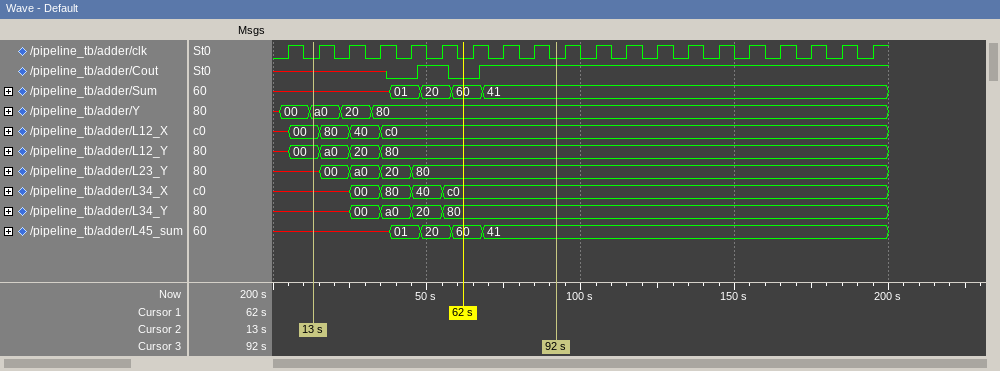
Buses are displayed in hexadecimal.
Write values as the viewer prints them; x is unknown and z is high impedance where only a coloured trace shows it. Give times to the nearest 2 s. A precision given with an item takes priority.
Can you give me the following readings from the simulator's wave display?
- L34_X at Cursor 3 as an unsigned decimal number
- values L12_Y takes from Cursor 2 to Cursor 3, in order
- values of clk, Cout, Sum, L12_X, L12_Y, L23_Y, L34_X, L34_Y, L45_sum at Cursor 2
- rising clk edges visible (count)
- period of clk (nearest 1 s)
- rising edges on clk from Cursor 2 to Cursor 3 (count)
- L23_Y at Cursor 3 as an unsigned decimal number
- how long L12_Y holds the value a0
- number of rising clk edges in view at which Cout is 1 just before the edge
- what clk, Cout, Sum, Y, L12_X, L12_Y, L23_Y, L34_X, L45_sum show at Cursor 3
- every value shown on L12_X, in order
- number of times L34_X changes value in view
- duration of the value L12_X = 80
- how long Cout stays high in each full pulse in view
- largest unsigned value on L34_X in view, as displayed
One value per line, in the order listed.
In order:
192
00, a0, 20, 80
clk=0, Cout=x, Sum=x, L12_X=00, L12_Y=00, L23_Y=x, L34_X=x, L34_Y=x, L45_sum=x
20
10 s
8
128
10 s
14
clk=0, Cout=1, Sum=41, Y=80, L12_X=c0, L12_Y=80, L23_Y=80, L34_X=c0, L45_sum=41
x, 00, 80, 40, c0
4
10 s
10 s
c0
